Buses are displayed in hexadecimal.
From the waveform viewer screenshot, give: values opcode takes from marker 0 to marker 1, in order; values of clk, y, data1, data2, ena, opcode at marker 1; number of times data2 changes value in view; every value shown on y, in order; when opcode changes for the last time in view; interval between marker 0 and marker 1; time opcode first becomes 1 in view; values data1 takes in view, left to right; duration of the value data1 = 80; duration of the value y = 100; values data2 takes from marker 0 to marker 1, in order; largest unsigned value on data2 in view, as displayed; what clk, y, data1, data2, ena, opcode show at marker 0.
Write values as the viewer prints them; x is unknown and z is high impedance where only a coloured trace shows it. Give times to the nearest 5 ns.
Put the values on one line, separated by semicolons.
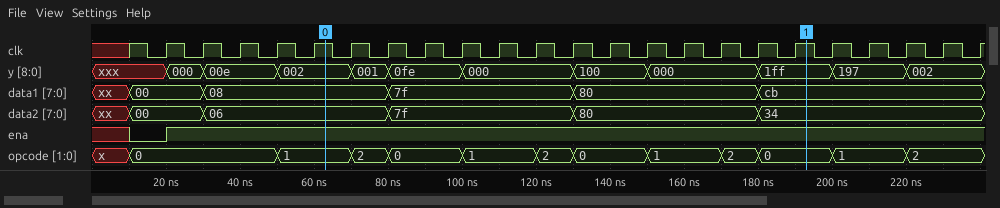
1, 2, 0, 1, 2, 0, 1, 2, 0; clk=1, y=1ff, data1=cb, data2=34, ena=1, opcode=0; 5; xxx, 000, 00e, 002, 001, 0fe, 000, 100, 000, 1ff, 197, 002; 220 ns; 130 ns; 50 ns; xx, 00, 08, 7f, 80, cb; 50 ns; 20 ns; 06, 7f, 80, 34; 80; clk=1, y=002, data1=08, data2=06, ena=1, opcode=1
